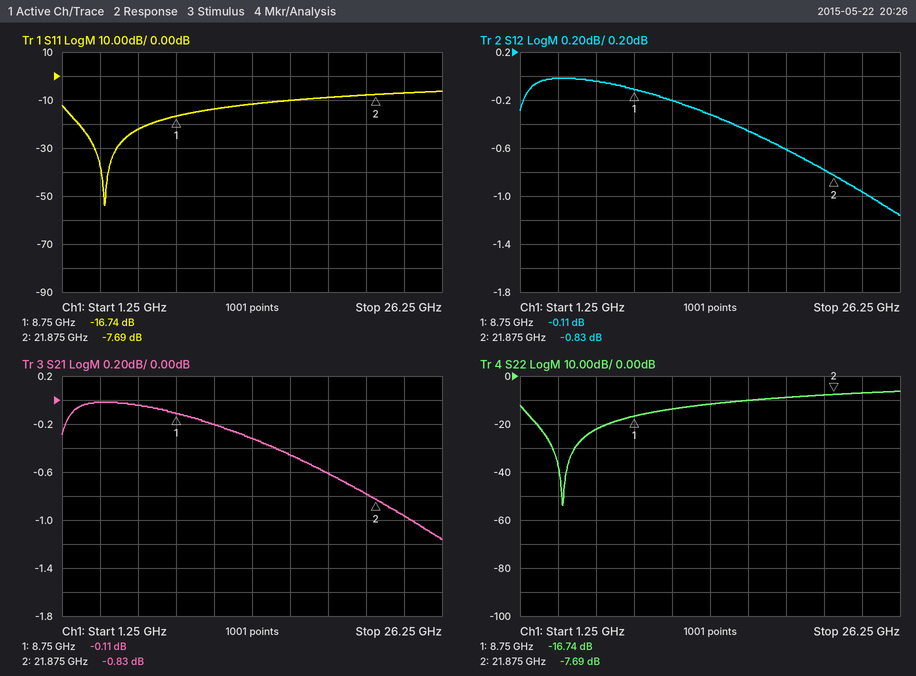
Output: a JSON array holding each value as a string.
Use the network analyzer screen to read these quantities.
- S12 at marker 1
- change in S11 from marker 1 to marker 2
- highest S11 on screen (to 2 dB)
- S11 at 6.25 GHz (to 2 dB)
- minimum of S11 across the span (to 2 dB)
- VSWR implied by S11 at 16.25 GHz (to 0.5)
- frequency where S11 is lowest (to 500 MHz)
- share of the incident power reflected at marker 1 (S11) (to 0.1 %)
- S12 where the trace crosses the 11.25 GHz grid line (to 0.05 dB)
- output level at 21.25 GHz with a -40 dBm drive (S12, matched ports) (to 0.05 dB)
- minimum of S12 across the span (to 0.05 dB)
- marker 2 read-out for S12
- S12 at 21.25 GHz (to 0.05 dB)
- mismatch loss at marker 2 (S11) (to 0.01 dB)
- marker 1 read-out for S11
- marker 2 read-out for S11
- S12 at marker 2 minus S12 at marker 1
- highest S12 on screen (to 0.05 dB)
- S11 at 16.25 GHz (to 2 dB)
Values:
["-0.11 dB", "9.05 dB", "-6 dB", "-22 dB", "-54 dB", "2.0", "4.0 GHz", "2.1 %", "-0.20 dB", "-40.80 dBm", "-1.15 dB", "-0.83 dB", "-0.80 dB", "0.81 dB", "-16.74 dB", "-7.69 dB", "-0.72 dB", "0.00 dB", "-10 dB"]
